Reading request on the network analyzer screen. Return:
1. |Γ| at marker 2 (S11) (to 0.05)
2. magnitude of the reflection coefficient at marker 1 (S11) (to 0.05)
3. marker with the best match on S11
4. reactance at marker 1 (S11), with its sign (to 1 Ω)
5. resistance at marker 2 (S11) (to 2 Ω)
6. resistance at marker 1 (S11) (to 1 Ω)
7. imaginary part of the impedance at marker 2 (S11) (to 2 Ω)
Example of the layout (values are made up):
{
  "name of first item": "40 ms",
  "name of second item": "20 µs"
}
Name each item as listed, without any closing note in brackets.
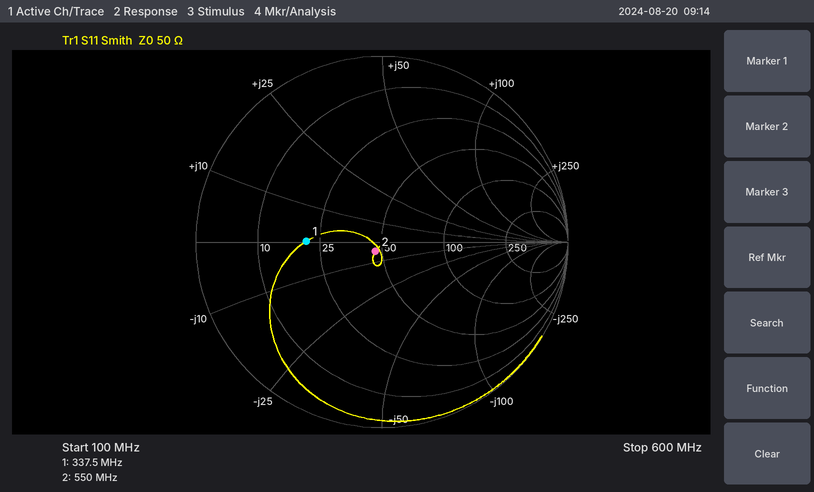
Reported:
{
  "|Γ| at marker 2 (S11)": "0.05",
  "magnitude of the reflection coefficient at marker 1 (S11)": "0.40",
  "marker with the best match on S11": "marker 2",
  "reactance at marker 1 (S11), with its sign": "0 Ω",
  "resistance at marker 2 (S11)": "46 Ω",
  "resistance at marker 1 (S11)": "21 Ω",
  "imaginary part of the impedance at marker 2 (S11)": "-4 Ω"
}
